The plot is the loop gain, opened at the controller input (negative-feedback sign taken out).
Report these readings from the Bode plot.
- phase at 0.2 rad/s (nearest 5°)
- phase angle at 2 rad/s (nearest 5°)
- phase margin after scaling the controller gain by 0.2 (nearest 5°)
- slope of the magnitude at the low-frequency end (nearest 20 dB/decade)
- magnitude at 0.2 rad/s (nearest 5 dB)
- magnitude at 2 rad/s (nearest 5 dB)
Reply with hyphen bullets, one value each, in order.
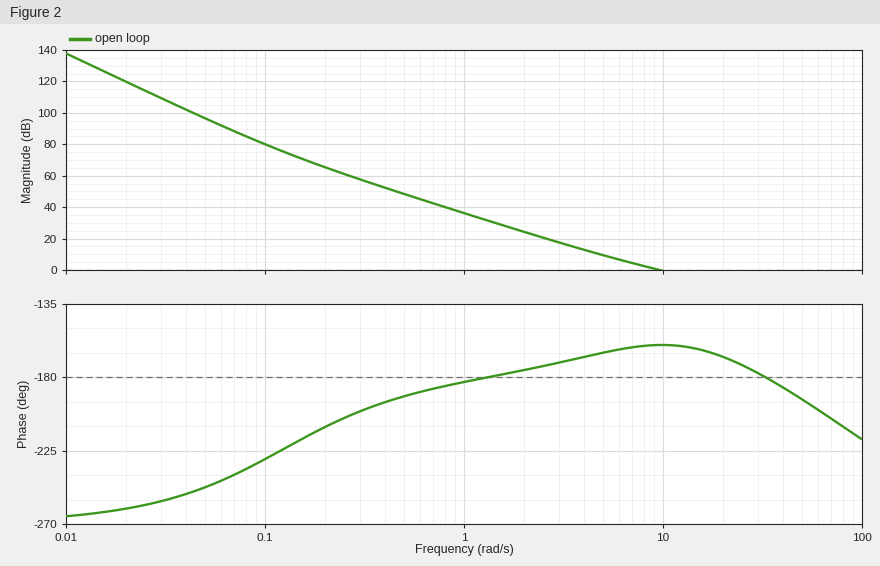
- -210°
- -175°
- 10°
- -60 dB/decade
- 65 dB
- 25 dB
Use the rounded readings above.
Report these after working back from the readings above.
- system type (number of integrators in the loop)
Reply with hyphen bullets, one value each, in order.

- 3
